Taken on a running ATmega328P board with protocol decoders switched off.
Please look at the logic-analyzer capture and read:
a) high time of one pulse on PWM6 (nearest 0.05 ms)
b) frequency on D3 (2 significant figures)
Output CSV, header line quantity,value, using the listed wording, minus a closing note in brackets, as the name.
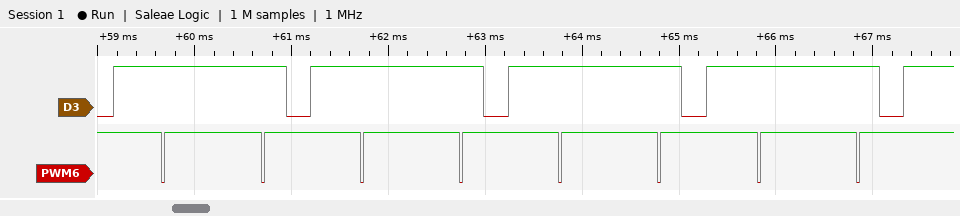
quantity,value
high time of one pulse on PWM6,1.00 ms
frequency on D3,490 Hz
